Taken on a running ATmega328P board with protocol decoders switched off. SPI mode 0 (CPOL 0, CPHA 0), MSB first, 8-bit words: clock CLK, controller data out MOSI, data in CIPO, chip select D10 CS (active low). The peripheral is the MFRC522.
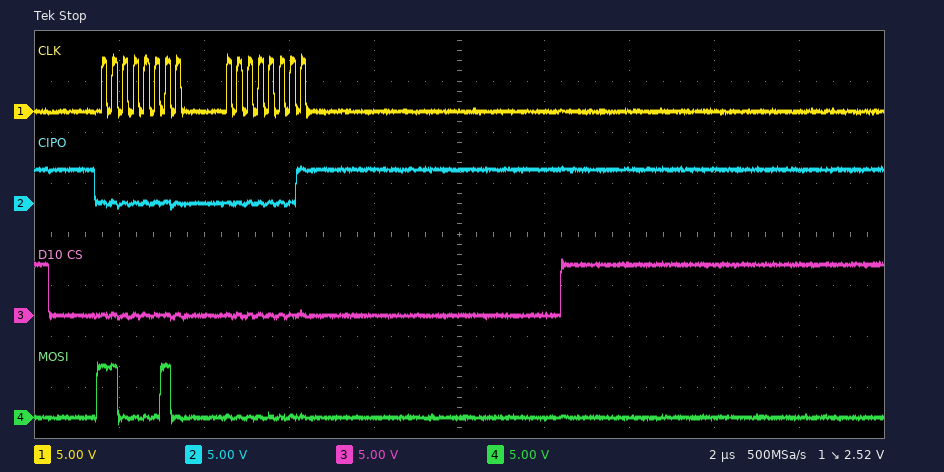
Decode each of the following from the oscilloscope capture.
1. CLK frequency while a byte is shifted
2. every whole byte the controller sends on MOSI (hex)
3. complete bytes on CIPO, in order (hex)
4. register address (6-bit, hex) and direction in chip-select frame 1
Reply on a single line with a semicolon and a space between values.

4 MHz; C2 00; 00 01; 0x21 read
